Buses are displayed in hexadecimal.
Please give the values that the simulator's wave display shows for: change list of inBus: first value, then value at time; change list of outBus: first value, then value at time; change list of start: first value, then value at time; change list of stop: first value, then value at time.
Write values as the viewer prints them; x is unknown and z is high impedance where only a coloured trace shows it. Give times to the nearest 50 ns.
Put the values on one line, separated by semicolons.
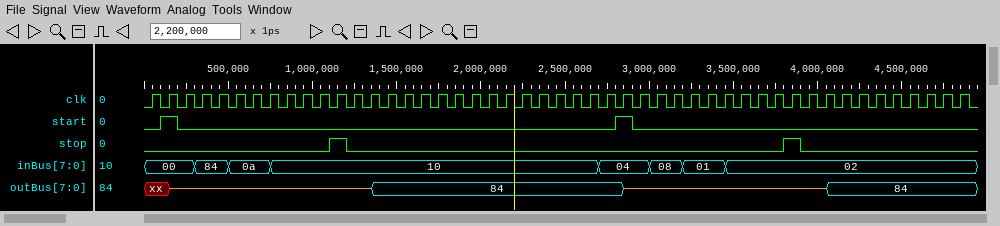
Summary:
00, 84 at 300 ns, 0a at 500 ns, 10 at 750 ns, 04 at 2700 ns, 08 at 3000 ns, 01 at 3200 ns, 02 at 3450 ns; xx, z at 150 ns, 84 at 1350 ns, z at 2850 ns, 84 at 4050 ns; 0, 1 at 100 ns, 0 at 200 ns, 1 at 2800 ns, 0 at 2900 ns; 0, 1 at 1100 ns, 0 at 1200 ns, 1 at 3800 ns, 0 at 3900 ns
